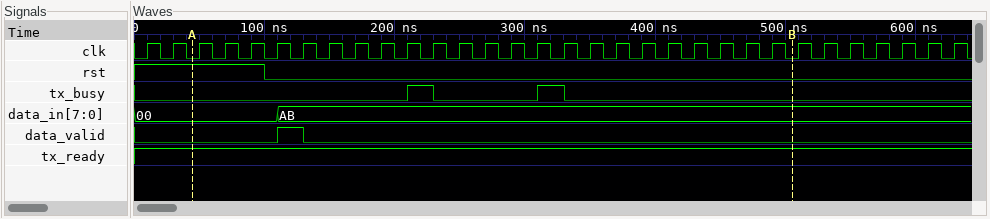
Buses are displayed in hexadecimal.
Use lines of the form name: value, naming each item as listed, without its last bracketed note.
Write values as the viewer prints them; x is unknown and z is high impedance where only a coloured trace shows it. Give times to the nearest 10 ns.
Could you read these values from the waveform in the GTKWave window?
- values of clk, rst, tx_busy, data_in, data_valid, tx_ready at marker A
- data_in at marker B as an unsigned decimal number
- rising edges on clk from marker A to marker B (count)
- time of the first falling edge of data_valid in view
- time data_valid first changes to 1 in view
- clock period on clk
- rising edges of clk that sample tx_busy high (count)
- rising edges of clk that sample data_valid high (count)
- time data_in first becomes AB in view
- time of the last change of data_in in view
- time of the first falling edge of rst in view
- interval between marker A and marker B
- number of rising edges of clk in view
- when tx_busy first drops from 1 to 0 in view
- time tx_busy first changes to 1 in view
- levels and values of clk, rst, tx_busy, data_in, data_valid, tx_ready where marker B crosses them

values of clk, rst, tx_busy, data_in, data_valid, tx_ready at marker A: clk=0, rst=1, tx_busy=0, data_in=00, data_valid=0, tx_ready=1
data_in at marker B as an unsigned decimal number: 171
rising edges on clk from marker A to marker B: 23
time of the first falling edge of data_valid in view: 130 ns
time data_valid first changes to 1 in view: 110 ns
clock period on clk: 20 ns
rising edges of clk that sample tx_busy high: 2
rising edges of clk that sample data_valid high: 1
time data_in first becomes AB in view: 110 ns
time of the last change of data_in in view: 110 ns
time of the first falling edge of rst in view: 100 ns
interval between marker A and marker B: 460 ns
number of rising edges of clk in view: 32
when tx_busy first drops from 1 to 0 in view: 230 ns
time tx_busy first changes to 1 in view: 210 ns
levels and values of clk, rst, tx_busy, data_in, data_valid, tx_ready where marker B crosses them: clk=0, rst=0, tx_busy=0, data_in=AB, data_valid=0, tx_ready=1
